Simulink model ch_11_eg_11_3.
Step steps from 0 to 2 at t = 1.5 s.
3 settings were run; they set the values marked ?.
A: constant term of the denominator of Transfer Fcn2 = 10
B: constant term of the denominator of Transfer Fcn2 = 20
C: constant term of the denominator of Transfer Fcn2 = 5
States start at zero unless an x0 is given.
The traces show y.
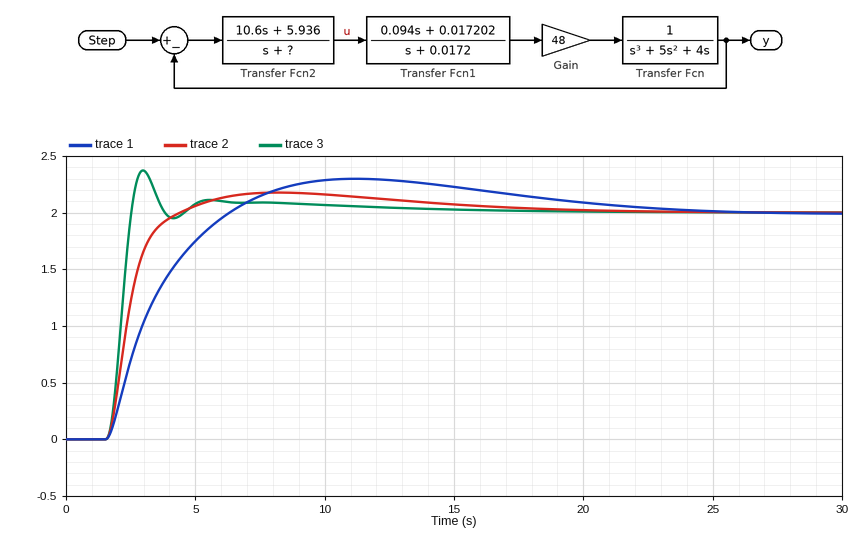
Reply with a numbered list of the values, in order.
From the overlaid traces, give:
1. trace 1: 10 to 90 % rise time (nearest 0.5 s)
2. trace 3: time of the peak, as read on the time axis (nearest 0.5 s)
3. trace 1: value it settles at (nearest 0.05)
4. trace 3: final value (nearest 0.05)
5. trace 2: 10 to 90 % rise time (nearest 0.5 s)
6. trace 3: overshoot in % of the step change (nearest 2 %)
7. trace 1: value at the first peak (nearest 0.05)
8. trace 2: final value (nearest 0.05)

1. 3.5 s
2. 3.0 s
3. 2.00
4. 2.00
5. 1.5 s
6. 18 %
7. 2.30
8. 2.00
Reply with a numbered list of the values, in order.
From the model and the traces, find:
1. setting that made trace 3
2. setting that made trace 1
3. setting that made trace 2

1. C
2. B
3. A
